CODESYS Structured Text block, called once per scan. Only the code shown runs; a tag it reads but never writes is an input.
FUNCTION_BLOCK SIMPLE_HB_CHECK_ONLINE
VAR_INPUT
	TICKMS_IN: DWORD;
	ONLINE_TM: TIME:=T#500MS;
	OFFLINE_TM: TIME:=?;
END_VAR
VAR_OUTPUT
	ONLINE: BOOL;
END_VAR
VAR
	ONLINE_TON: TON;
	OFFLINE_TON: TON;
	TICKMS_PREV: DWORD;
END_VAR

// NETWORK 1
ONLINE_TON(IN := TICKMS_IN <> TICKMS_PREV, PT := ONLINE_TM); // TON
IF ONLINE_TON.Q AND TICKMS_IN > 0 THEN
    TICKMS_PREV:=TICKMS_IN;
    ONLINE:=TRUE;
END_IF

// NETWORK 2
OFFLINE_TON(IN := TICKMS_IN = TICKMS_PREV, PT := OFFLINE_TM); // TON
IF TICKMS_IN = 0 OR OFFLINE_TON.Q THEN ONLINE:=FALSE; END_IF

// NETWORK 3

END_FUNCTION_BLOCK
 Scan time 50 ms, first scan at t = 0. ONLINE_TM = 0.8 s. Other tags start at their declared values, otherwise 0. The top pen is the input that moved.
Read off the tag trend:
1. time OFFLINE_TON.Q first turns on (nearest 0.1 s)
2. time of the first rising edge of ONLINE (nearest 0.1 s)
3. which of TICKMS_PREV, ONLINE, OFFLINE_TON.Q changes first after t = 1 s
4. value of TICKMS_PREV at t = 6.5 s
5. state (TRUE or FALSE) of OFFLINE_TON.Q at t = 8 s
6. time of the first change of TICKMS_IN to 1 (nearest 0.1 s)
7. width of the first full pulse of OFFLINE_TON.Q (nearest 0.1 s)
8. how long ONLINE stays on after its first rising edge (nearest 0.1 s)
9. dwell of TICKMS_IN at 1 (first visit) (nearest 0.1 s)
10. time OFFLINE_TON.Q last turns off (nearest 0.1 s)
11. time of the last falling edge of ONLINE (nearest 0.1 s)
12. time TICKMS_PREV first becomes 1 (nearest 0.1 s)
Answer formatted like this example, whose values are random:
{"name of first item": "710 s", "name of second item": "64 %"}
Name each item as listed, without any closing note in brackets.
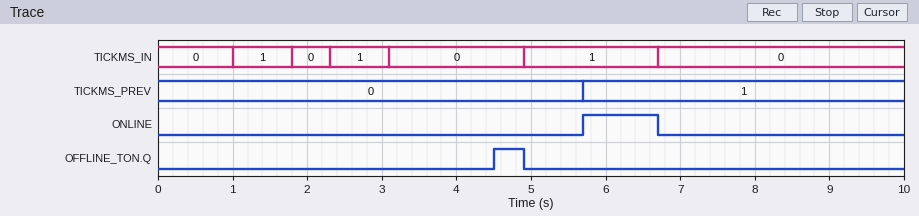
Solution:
{"time OFFLINE_TON.Q first turns on": "4.5 s", "time of the first rising edge of ONLINE": "5.7 s", "which of TICKMS_PREV, ONLINE, OFFLINE_TON.Q changes first after t = 1 s": "OFFLINE_TON.Q", "value of TICKMS_PREV at t = 6.5 s": "1", "state (TRUE or FALSE) of OFFLINE_TON.Q at t = 8 s": "FALSE", "time of the first change of TICKMS_IN to 1": "1.0 s", "width of the first full pulse of OFFLINE_TON.Q": "0.4 s", "how long ONLINE stays on after its first rising edge": "1.0 s", "dwell of TICKMS_IN at 1 (first visit)": "0.8 s", "time OFFLINE_TON.Q last turns off": "4.9 s", "time of the last falling edge of ONLINE": "6.7 s", "time TICKMS_PREV first becomes 1": "5.7 s"}
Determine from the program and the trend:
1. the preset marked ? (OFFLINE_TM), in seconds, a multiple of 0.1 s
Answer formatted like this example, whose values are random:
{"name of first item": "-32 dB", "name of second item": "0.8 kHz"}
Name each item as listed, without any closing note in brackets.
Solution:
{"the preset marked ? (OFFLINE_TM), in seconds, a multiple of 0.1 s": "1.4 s"}
